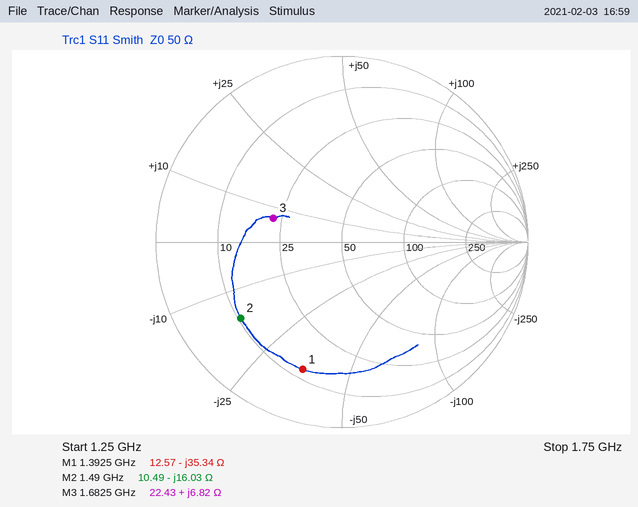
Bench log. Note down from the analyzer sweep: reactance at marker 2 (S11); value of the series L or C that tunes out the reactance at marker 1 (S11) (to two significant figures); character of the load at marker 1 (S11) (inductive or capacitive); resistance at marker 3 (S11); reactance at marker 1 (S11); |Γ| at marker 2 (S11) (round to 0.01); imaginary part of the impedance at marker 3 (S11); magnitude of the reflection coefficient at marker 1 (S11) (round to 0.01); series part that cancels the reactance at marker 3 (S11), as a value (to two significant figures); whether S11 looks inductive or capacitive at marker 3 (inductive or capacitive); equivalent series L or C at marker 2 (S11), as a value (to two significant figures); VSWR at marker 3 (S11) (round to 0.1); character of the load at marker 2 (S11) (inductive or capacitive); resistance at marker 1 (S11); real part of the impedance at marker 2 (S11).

-16.03 Ω
4.0 nH
capacitive
22.43 Ω
-35.34 Ω
0.68
+6.82 Ω
0.72
14 pF
inductive
6.7 pF
2.3
capacitive
12.57 Ω
10.49 Ω
